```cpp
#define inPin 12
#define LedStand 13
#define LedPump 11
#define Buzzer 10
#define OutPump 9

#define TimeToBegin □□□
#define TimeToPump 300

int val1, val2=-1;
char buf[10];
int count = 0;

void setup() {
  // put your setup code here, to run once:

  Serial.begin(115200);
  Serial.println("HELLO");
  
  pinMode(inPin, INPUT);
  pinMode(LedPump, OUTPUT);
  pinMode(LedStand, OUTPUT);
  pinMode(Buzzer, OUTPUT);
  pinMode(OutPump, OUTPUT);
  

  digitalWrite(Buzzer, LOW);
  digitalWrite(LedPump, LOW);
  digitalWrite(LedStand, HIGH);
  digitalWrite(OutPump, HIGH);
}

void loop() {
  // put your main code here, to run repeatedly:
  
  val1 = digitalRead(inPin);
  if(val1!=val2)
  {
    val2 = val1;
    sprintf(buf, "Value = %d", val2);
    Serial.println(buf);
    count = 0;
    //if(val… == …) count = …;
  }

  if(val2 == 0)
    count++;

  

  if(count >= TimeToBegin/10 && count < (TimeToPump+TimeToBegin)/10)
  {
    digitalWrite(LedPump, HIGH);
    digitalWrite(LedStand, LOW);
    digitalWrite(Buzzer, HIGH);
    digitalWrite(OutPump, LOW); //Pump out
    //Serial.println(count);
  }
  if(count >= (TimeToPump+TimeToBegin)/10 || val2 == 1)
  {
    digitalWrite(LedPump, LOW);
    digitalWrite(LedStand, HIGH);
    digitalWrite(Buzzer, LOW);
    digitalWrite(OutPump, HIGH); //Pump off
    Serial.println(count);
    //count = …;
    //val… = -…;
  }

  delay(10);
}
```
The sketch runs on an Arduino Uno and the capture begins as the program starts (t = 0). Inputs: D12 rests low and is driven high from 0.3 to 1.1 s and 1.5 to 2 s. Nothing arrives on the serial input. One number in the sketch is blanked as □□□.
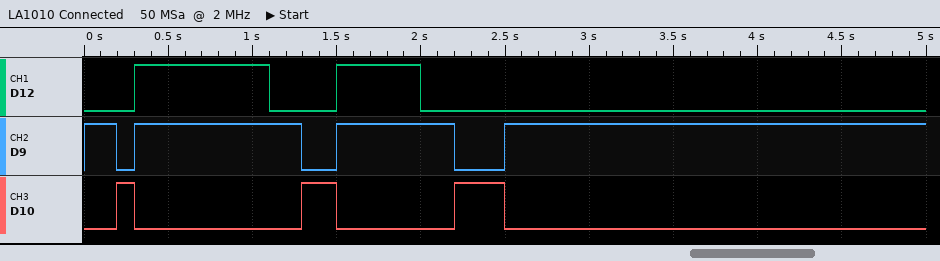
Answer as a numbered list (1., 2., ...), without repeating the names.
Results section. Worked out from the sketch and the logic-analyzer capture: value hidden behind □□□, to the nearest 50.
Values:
1. 200
